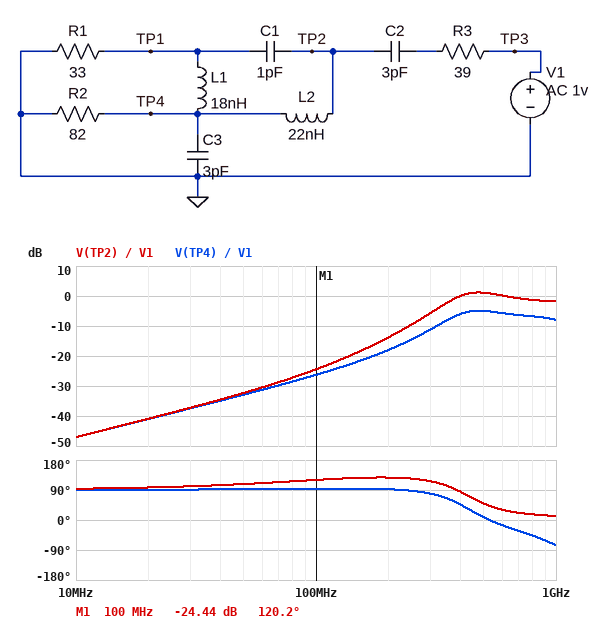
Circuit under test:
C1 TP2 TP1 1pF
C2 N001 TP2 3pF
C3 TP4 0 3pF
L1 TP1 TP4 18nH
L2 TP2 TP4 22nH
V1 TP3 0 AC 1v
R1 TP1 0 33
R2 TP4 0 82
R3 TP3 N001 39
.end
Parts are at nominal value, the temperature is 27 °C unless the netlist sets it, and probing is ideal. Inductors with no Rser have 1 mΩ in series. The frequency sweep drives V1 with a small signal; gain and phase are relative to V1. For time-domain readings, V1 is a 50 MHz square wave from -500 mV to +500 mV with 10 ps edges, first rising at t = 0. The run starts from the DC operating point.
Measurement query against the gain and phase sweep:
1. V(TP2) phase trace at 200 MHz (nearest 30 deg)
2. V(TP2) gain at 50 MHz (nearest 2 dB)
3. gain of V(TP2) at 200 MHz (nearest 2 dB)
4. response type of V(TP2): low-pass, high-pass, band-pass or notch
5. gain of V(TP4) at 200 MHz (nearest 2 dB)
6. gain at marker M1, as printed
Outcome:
120 deg
-32 dB
-14 dB
high-pass
-18 dB
-24.44 dB
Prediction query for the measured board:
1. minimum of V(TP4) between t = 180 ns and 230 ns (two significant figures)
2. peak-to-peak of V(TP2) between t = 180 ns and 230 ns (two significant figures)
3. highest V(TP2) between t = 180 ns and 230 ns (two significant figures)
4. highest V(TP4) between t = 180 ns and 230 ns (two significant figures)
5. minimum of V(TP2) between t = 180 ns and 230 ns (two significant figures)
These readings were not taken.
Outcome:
-270 mV
1.2 V
610 mV
270 mV
-610 mV
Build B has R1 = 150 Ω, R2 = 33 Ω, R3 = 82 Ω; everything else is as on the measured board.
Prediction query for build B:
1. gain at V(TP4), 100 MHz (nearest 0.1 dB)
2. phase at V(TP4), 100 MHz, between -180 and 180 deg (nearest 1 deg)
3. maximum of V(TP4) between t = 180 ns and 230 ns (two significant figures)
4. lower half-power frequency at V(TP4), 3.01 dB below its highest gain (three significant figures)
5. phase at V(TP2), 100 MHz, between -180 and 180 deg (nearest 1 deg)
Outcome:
-25.8 dB
76 deg
140 mV
338 MHz
104 deg
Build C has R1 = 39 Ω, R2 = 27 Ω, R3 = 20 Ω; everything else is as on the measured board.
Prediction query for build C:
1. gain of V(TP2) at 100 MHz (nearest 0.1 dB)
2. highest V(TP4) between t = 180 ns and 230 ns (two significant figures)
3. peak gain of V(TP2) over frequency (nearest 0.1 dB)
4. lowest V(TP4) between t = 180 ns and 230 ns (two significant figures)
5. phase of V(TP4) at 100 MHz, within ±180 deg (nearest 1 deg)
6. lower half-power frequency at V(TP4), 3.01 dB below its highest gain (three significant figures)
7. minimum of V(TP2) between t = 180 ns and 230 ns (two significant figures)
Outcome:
-27.2 dB
150 mV
5.4 dB
-150 mV
91 deg
420 MHz
-680 mV
